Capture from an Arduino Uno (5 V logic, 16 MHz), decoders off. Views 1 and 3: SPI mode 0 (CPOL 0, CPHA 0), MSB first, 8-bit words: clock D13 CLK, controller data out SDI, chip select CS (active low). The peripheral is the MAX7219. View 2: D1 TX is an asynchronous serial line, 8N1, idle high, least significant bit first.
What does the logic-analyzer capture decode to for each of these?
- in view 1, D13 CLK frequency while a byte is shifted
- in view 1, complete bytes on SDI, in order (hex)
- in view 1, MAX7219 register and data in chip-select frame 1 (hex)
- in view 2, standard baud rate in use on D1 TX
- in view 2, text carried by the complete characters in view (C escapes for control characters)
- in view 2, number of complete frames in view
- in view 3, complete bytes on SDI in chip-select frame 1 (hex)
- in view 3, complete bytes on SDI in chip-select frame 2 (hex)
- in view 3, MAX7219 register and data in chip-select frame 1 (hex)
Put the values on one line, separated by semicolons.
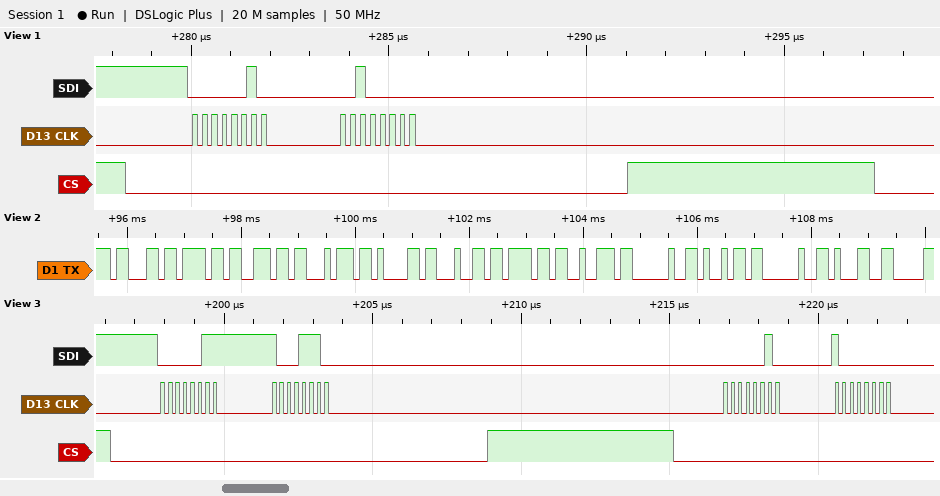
4 MHz; 02 20; register 0x2, data 0x20; 9600 baud; "contador i 1"; 12; 0x03 0x8E; 0x02 0x80; register 0x3, data 0x8E
